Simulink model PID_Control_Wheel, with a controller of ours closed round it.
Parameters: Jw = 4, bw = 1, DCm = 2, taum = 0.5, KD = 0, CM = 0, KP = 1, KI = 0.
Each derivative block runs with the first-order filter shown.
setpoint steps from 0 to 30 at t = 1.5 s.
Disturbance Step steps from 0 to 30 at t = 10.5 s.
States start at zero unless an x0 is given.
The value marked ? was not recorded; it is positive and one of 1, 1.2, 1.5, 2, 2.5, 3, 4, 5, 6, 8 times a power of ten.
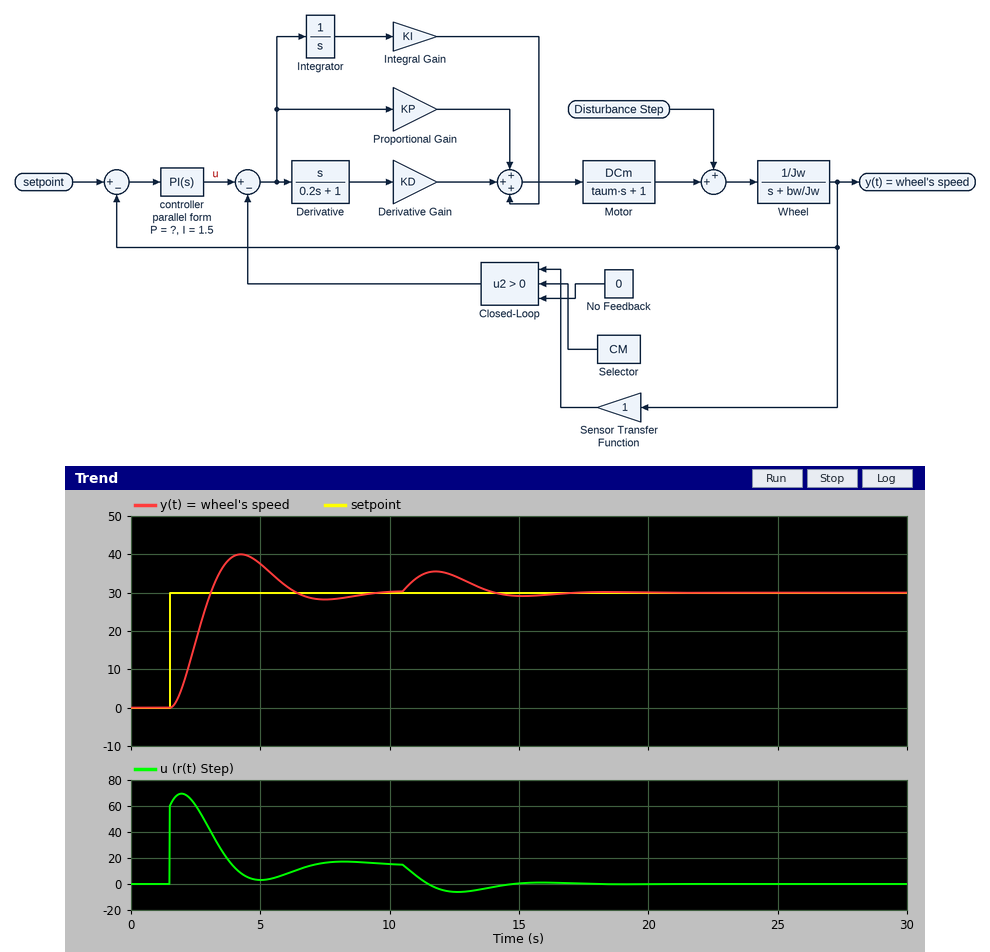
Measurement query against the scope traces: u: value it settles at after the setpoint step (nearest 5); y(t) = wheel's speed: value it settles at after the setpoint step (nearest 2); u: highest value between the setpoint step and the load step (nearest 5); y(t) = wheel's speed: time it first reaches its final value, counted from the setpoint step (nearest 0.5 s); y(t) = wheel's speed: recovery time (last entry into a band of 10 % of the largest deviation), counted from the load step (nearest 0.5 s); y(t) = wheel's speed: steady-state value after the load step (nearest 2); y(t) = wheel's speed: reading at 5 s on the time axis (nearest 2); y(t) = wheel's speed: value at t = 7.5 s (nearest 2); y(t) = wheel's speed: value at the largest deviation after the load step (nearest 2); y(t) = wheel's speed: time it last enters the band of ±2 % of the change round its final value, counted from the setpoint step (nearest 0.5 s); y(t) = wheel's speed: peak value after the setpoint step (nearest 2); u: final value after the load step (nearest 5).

15
30
70
1.5 s
5.5 s
30
38
28
36
7.5 s
40
0
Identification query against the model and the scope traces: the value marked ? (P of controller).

2
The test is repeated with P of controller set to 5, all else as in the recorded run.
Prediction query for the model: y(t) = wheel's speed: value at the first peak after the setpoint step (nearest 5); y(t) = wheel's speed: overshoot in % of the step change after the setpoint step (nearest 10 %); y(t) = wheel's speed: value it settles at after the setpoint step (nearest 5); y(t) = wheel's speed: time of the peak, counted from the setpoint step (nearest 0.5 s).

35
20 %
30
1.5 s
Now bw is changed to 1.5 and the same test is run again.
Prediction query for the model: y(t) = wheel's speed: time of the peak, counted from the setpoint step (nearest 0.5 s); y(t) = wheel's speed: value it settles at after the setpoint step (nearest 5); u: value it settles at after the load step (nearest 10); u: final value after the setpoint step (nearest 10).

3.0 s
30
10
20
